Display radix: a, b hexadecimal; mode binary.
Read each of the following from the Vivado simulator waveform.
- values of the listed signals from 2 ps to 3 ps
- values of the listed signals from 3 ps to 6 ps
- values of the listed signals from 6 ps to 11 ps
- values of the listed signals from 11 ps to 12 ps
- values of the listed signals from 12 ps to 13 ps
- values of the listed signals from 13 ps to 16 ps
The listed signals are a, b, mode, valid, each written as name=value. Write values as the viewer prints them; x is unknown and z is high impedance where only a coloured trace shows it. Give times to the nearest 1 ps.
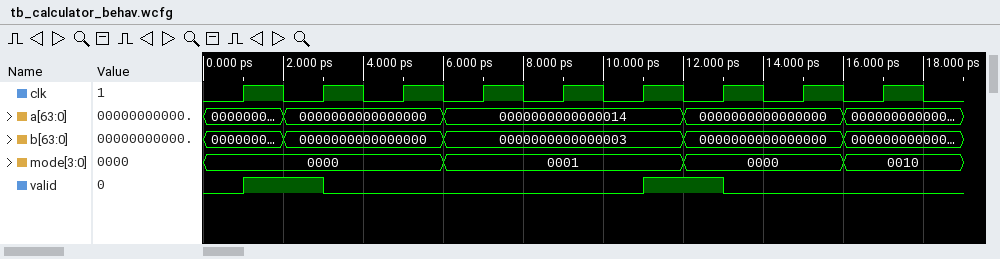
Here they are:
a=0000000000000000, b=0000000000000000, mode=0000, valid=1
a=0000000000000000, b=0000000000000000, mode=0000, valid=0
a=0000000000000014, b=0000000000000003, mode=0001, valid=0
a=0000000000000014, b=0000000000000003, mode=0001, valid=1
a=0000000000000000, b=0000000000000000, mode=0000, valid=1
a=0000000000000000, b=0000000000000000, mode=0000, valid=0
